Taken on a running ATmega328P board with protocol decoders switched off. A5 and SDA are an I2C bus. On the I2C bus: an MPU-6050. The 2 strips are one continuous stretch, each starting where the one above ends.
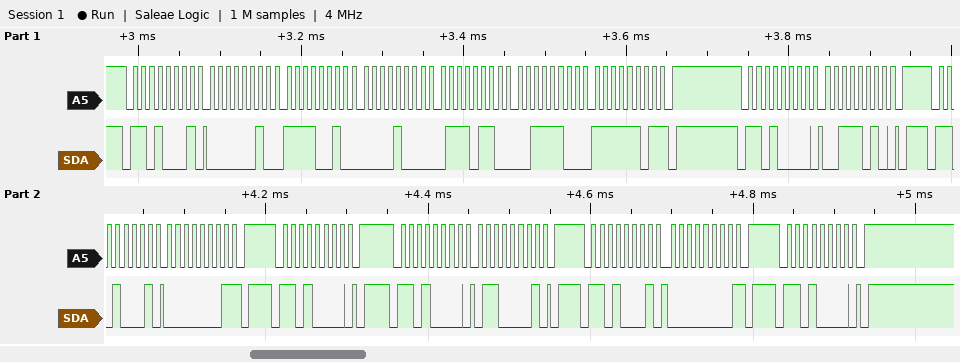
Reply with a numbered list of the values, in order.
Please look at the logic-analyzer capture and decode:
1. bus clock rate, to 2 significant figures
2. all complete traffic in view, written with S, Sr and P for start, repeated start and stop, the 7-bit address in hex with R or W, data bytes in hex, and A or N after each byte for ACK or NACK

1. 100 kHz
2. S 68R A 02 A F2 A 08 A 76 A 3C A FD N P S 68W A 3A A P S 68R A 01 N P S 68W A P S 68W A 61 A P S 68R A 00 N P S 68W A P
